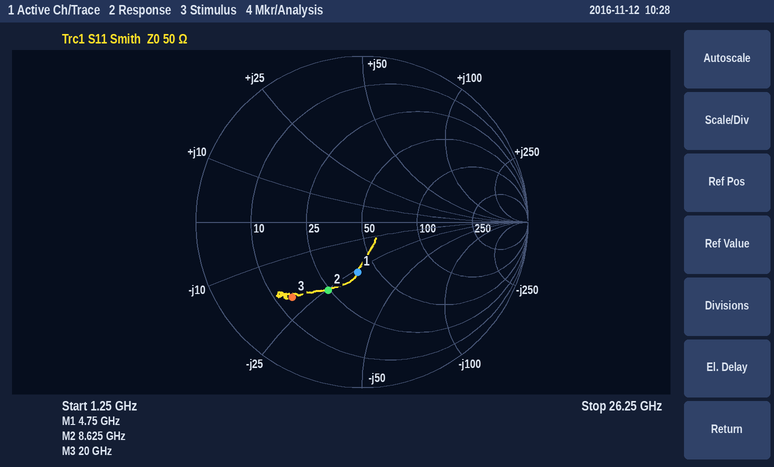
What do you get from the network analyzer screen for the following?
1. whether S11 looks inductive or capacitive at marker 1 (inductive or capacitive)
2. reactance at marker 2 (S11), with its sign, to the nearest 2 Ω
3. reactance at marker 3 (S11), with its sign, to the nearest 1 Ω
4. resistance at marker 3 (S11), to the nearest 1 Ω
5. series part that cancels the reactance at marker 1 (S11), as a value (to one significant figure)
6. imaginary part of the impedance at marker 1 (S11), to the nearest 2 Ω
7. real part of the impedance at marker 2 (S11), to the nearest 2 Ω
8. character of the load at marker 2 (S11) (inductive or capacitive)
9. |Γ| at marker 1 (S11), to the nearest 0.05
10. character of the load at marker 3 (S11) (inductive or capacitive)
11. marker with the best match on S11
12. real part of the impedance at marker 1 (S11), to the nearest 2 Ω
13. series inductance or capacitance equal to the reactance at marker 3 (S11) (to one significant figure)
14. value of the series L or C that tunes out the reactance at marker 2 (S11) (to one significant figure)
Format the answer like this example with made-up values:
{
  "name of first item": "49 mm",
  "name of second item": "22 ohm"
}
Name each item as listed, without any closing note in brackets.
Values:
{
  "whether S11 looks inductive or capacitive at marker 1": "capacitive",
  "reactance at marker 2 (S11), with its sign, to the nearest 2 Ω": "-26 Ω",
  "reactance at marker 3 (S11), with its sign, to the nearest 1 Ω": "-20 Ω",
  "resistance at marker 3 (S11), to the nearest 1 Ω": "14 Ω",
  "series part that cancels the reactance at marker 1 (S11), as a value": "900 pH",
  "imaginary part of the impedance at marker 1 (S11), to the nearest 2 Ω": "-26 Ω",
  "real part of the impedance at marker 2 (S11), to the nearest 2 Ω": "24 Ω",
  "character of the load at marker 2 (S11)": "capacitive",
  "|Γ| at marker 1 (S11), to the nearest 0.05": "0.30",
  "character of the load at marker 3 (S11)": "capacitive",
  "marker with the best match on S11": "marker 1",
  "real part of the impedance at marker 1 (S11), to the nearest 2 Ω": "40 Ω",
  "series inductance or capacitance equal to the reactance at marker 3 (S11)": "400 fF",
  "value of the series L or C that tunes out the reactance at marker 2 (S11)": "500 pH"
}
